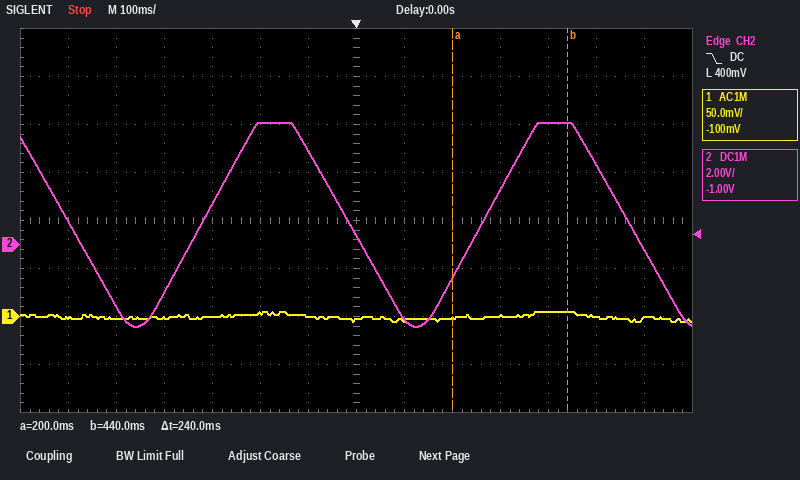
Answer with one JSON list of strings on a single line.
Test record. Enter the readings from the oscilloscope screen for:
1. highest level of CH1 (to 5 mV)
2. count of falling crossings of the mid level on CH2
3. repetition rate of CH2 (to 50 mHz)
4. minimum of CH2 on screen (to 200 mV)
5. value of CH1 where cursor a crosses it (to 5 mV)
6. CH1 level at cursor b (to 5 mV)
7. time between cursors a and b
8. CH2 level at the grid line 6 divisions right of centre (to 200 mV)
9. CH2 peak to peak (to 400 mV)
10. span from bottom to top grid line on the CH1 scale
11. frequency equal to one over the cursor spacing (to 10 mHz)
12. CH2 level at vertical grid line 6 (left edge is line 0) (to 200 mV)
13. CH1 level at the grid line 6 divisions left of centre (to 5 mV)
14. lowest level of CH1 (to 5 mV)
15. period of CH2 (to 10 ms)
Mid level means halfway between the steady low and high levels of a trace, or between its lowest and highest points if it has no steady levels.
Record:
["5 mV", "3", "1.70 Hz", "-3.4 V", "0 mV", "5 mV", "240 ms", "-200 mV", "8.4 V", "400 mV", "4.17 Hz", "4.0 V", "0 mV", "-5 mV", "580 ms"]
